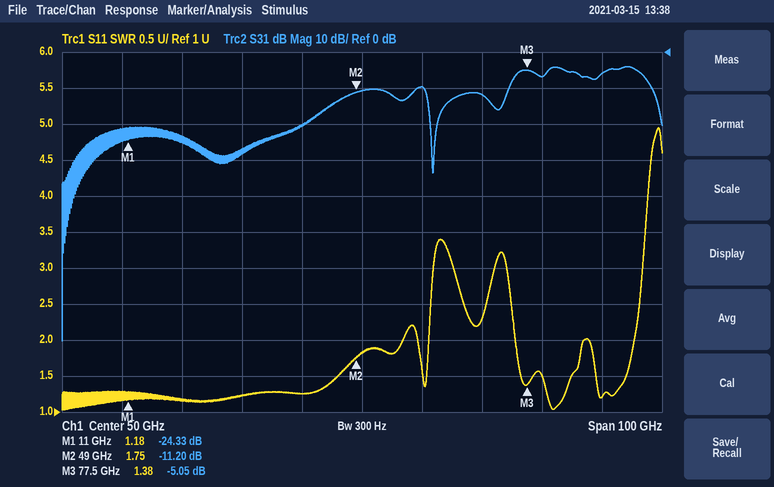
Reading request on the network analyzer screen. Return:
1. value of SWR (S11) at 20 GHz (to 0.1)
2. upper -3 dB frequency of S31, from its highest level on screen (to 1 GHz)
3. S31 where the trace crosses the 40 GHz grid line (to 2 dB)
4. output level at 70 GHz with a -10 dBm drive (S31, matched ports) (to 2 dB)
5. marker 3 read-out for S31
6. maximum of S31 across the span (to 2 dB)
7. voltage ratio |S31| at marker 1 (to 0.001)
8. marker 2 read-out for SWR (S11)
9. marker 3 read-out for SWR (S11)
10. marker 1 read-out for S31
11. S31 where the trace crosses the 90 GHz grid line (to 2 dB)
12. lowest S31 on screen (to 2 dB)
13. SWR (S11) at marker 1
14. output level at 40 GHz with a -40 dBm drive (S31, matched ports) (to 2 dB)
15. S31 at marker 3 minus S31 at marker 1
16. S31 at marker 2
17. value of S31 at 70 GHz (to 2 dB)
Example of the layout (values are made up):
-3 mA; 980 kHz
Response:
1.2; 97 GHz; -20 dB; -22 dBm; -5.05 dB; -4 dB; 0.061; 1.75; 1.38; -24.33 dB; -6 dB; -80 dB; 1.18; -60 dBm; 19.28 dB; -11.20 dB; -12 dB
